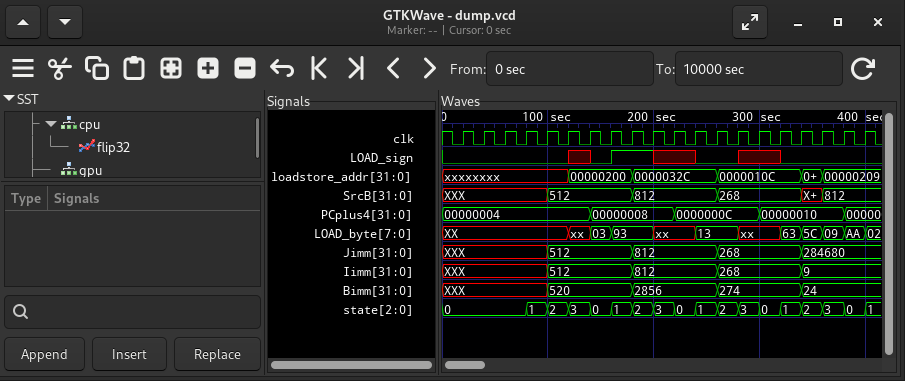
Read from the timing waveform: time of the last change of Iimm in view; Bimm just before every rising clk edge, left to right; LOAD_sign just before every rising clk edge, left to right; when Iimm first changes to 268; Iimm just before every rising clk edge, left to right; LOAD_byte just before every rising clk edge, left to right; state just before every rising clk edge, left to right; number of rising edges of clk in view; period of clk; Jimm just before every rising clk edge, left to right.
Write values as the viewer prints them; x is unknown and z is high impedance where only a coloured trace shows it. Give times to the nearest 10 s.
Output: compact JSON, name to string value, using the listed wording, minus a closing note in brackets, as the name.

{"time of the last change of Iimm in view": "340 s", "Bimm just before every rising clk edge, left to right": "XXX, XXX, XXX, XXX, XXX, 520, 520, 520, 520, 2856, 2856, 2856, 2856, 274, 274, 274, 274, 24, 24, 24", "LOAD_sign just before every rising clk edge, left to right": "0 0 0 0 0 0 x 0 1 1 x x 0 0 x x 0 0 0 0", "when Iimm first changes to 268": "260 s", "Iimm just before every rising clk edge, left to right": "XXX, XXX, XXX, XXX, XXX, 512, 512, 512, 512, 812, 812, 812, 812, 268, 268, 268, 268, 9, 9, 9", "LOAD_byte just before every rising clk edge, left to right": "XX, XX, XX, XX, XX, XX, xx, 03, 93, 93, xx, xx, 13, 13, xx, xx, 63, 5C, 09, AA", "state just before every rising clk edge, left to right": "0, 0, 0, 0, 1, 2, 3, 0, 1, 2, 3, 0, 1, 2, 3, 0, 1, 2, 3, 0", "number of rising edges of clk in view": "20", "period of clk": "20 s", "Jimm just before every rising clk edge, left to right": "XXX, XXX, XXX, XXX, XXX, 512, 512, 512, 512, 812, 812, 812, 812, 268, 268, 268, 268, 284680, 284680, 284680"}
